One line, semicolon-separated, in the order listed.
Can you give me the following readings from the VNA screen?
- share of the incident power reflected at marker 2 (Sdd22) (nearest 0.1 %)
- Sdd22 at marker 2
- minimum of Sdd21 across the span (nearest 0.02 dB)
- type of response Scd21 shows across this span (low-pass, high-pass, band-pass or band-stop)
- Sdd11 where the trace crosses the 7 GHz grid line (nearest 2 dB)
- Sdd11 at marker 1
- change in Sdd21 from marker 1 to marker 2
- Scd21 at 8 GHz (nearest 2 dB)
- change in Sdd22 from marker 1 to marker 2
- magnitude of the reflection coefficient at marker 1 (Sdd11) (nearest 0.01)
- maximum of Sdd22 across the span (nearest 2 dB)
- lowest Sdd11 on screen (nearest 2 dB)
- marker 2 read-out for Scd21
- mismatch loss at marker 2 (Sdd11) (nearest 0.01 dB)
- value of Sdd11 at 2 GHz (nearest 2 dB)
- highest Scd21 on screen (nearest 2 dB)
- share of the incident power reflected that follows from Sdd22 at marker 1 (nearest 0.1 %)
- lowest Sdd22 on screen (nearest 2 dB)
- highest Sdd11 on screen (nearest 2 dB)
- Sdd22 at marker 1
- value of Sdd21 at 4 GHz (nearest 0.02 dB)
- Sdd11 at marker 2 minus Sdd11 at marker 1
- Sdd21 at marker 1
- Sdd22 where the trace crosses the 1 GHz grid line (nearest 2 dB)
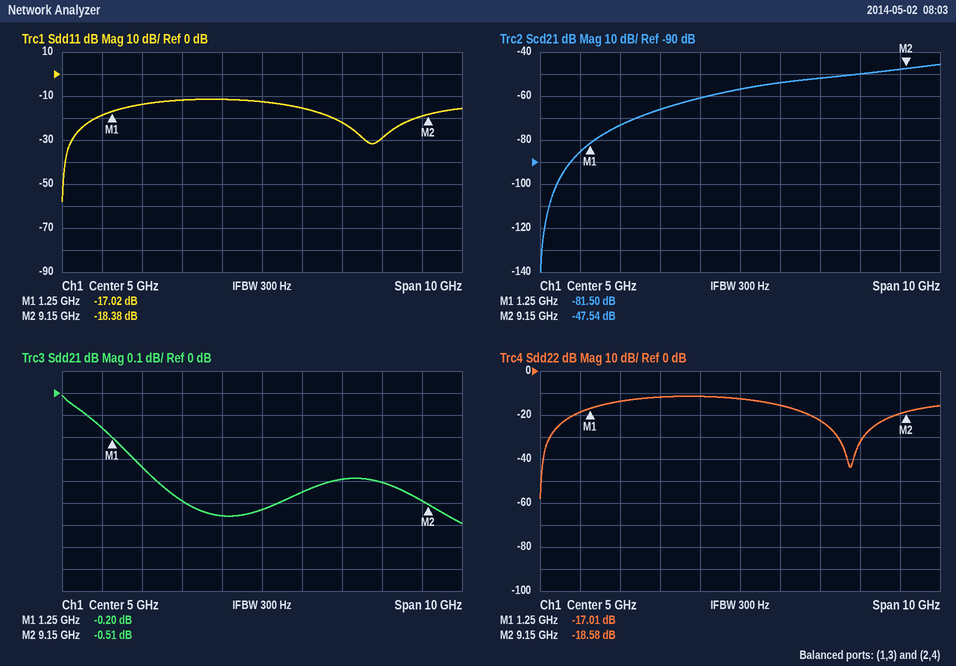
1.4 %; -18.58 dB; -0.60 dB; high-pass; -22 dB; -17.02 dB; -0.31 dB; -50 dB; -1.57 dB; 0.14; -12 dB; -58 dB; -47.54 dB; 0.06 dB; -14 dB; -46 dB; 2.0 %; -58 dB; -12 dB; -17.01 dB; -0.56 dB; -1.36 dB; -0.20 dB; -18 dB
